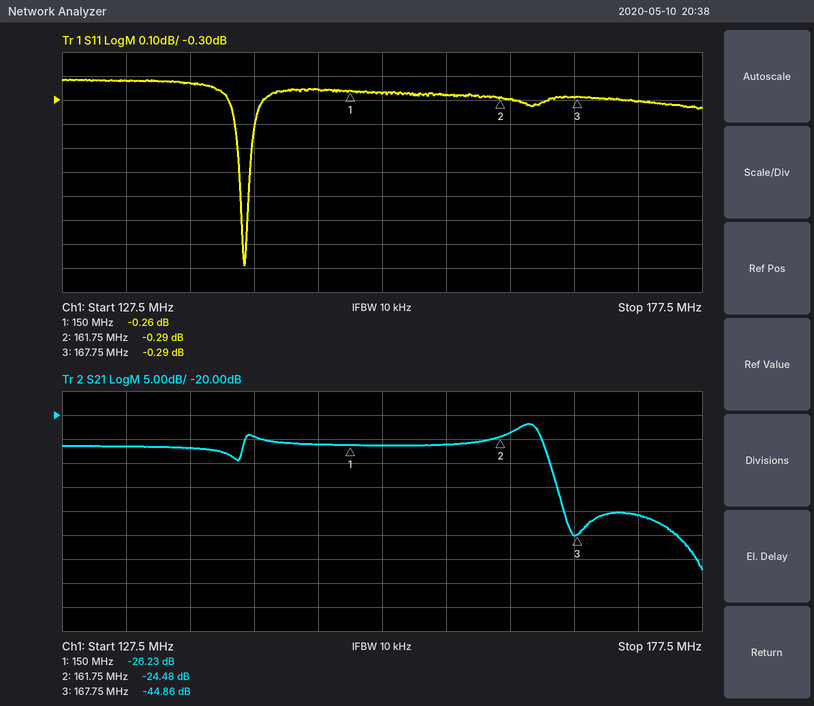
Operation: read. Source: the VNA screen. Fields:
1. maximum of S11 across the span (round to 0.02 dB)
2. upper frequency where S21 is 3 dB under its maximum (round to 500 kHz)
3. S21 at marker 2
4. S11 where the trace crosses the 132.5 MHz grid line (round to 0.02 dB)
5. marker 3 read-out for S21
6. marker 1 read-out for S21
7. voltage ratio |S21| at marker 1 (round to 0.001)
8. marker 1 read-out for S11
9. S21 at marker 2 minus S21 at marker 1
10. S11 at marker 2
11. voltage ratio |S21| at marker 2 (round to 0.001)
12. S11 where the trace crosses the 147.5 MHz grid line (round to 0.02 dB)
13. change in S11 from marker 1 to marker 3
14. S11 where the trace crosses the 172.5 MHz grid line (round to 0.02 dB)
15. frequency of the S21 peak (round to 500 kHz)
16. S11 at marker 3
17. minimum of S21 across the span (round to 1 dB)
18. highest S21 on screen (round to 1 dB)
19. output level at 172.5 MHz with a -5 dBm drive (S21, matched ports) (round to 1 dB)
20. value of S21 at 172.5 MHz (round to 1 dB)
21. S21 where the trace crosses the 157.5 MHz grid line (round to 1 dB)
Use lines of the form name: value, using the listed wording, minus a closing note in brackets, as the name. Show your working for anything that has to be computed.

maximum of S11 across the span: -0.22 dB
upper frequency where S21 is 3 dB under its maximum: 165.0 MHz
S21 at marker 2: -24.48 dB
S11 where the trace crosses the 132.5 MHz grid line: -0.22 dB
marker 3 read-out for S21: -44.86 dB
marker 1 read-out for S21: -26.23 dB
voltage ratio |S21| at marker 1: 10^(-26.23/20) ≈ 0.049
marker 1 read-out for S11: -0.26 dB
S21 at marker 2 minus S21 at marker 1: -24.48 − (-26.23) = 1.75 dB
S11 at marker 2: -0.29 dB
voltage ratio |S21| at marker 2: 10^(-24.48/20) ≈ 0.060
S11 where the trace crosses the 147.5 MHz grid line: -0.26 dB
change in S11 from marker 1 to marker 3: -0.29 − (-0.26) = -0.03 dB
S11 where the trace crosses the 172.5 MHz grid line: -0.30 dB
frequency of the S21 peak: 164.0 MHz
S11 at marker 3: -0.29 dB
minimum of S21 across the span: -52 dB
highest S21 on screen: -22 dB
output level at 172.5 MHz with a -5 dBm drive (S21, matched ports): -5 dBm + (-41 dB) = -46 dBm
value of S21 at 172.5 MHz: -41 dB
S21 where the trace crosses the 157.5 MHz grid line: -26 dB
